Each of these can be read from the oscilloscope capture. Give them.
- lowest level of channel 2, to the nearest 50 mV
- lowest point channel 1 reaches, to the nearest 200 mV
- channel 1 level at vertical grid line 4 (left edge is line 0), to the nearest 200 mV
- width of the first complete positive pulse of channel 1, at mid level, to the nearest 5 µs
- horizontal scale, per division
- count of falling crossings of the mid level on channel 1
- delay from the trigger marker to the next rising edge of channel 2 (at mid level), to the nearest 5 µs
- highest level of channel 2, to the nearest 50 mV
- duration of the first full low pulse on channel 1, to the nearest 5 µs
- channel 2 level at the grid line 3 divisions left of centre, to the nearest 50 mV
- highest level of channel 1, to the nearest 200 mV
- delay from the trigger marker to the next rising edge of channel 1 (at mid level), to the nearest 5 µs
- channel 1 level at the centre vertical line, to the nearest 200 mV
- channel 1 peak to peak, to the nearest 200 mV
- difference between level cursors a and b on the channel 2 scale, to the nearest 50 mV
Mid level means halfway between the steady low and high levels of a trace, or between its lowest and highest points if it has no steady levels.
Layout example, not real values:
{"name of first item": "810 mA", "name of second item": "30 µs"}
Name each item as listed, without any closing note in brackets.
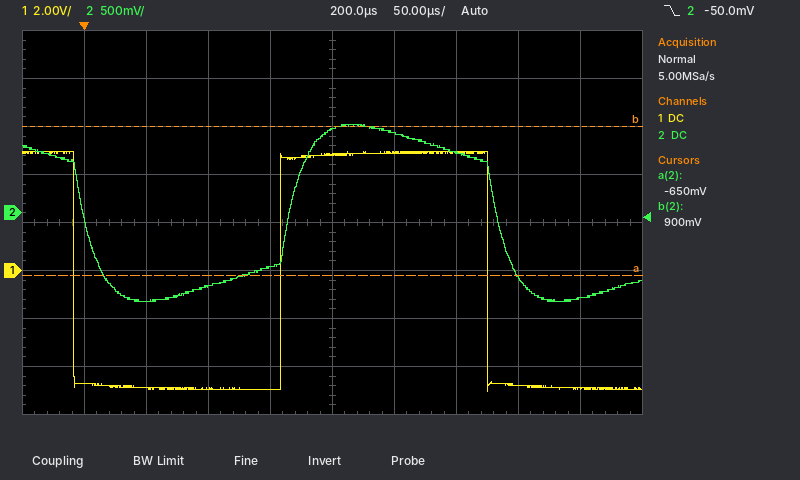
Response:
{"lowest level of channel 2, to the nearest 50 mV": "-900 mV", "lowest point channel 1 reaches, to the nearest 200 mV": "-5.0 V", "channel 1 level at vertical grid line 4 (left edge is line 0), to the nearest 200 mV": "-5.0 V", "width of the first complete positive pulse of channel 1, at mid level, to the nearest 5 µs": "165 µs", "horizontal scale, per division": "50 µs", "count of falling crossings of the mid level on channel 1": "2", "delay from the trigger marker to the next rising edge of channel 2 (at mid level), to the nearest 5 µs": "165 µs", "highest level of channel 2, to the nearest 50 mV": "900 mV", "duration of the first full low pulse on channel 1, to the nearest 5 µs": "165 µs", "channel 2 level at the grid line 3 divisions left of centre, to the nearest 50 mV": "-900 mV", "highest level of channel 1, to the nearest 200 mV": "5.0 V", "delay from the trigger marker to the next rising edge of channel 1 (at mid level), to the nearest 5 µs": "160 µs", "channel 1 level at the centre vertical line, to the nearest 200 mV": "4.8 V", "channel 1 peak to peak, to the nearest 200 mV": "10.0 V", "difference between level cursors a and b on the channel 2 scale, to the nearest 50 mV": "1.55 V"}
